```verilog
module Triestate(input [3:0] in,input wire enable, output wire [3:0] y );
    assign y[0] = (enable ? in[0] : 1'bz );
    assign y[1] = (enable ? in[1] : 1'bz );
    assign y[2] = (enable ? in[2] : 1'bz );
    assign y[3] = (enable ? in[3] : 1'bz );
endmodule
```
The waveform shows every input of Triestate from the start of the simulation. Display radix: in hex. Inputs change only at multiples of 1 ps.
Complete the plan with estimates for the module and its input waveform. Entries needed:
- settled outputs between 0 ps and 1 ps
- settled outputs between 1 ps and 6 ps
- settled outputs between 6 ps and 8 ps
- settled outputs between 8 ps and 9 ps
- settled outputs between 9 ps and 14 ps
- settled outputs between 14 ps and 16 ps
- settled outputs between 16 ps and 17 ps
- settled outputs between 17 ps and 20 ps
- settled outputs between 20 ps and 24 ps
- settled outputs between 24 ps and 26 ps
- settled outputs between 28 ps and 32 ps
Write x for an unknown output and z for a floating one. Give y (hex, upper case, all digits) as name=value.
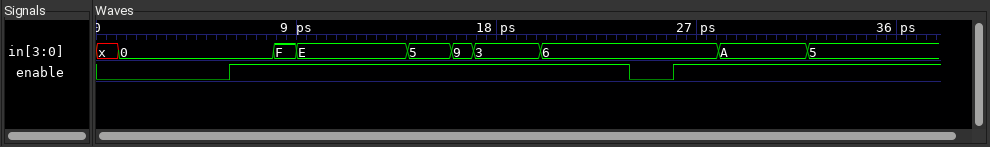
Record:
y=z
y=z
y=0
y=F
y=E
y=5
y=9
y=3
y=6
y=z
y=A
